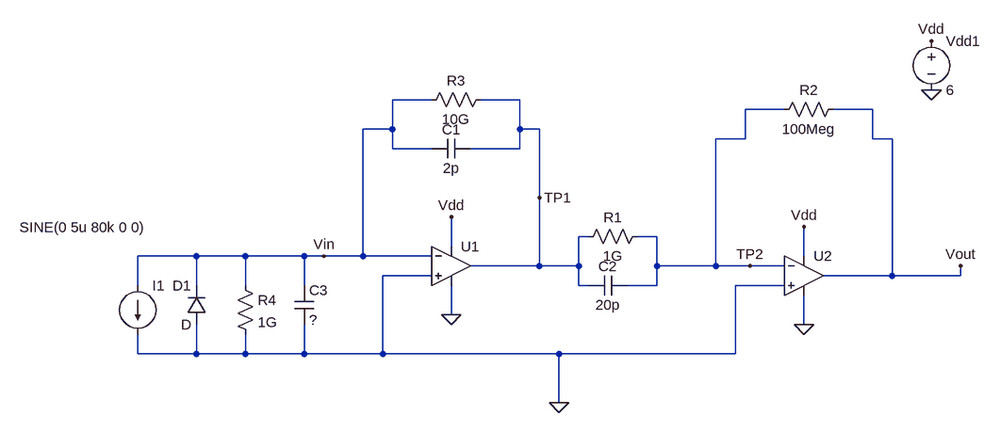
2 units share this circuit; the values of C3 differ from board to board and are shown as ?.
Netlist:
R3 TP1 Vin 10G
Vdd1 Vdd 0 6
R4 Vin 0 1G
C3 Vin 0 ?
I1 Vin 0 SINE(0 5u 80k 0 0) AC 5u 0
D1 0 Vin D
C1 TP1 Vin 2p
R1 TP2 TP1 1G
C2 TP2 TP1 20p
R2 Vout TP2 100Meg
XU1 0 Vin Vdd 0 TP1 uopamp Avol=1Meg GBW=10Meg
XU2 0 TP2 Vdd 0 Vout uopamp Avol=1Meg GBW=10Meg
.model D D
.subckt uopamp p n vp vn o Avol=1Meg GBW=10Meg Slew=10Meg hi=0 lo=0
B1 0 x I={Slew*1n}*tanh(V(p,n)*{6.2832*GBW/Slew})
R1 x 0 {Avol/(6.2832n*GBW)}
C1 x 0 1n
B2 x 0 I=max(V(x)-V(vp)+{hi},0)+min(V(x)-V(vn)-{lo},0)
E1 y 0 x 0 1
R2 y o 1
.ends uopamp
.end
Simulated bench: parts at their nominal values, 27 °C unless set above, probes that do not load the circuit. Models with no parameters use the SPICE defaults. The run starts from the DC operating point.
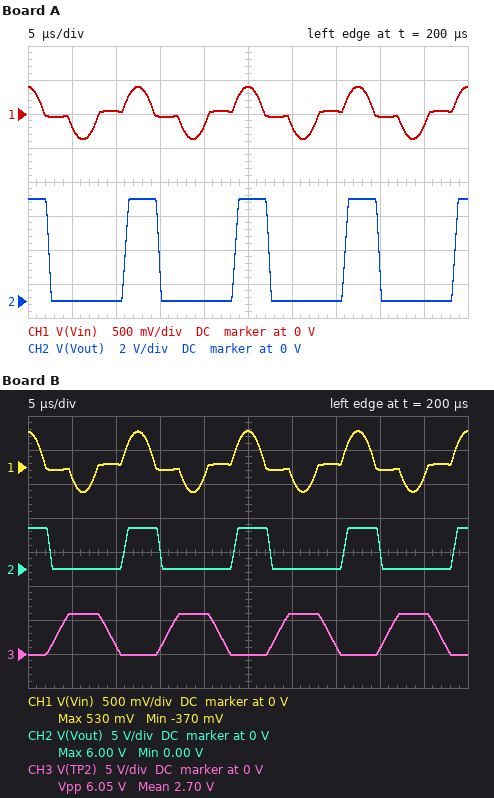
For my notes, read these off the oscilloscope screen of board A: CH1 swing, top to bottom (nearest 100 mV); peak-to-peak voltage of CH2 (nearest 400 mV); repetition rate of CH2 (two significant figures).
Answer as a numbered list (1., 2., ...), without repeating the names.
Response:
1. 800 mV
2. 6.0 V
3. 80 kHz
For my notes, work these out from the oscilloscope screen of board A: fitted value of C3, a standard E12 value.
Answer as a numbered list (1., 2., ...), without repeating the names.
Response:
1. 8.2 pF
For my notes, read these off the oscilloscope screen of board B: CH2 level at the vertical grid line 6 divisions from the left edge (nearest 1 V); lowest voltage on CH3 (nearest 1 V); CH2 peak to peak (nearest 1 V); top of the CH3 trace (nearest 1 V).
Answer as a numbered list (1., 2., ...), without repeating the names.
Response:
1. 0 V
2. 0 V
3. 6 V
4. 6 V
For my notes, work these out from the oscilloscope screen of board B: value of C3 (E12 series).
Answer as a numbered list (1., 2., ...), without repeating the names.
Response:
1. 6.8 pF
